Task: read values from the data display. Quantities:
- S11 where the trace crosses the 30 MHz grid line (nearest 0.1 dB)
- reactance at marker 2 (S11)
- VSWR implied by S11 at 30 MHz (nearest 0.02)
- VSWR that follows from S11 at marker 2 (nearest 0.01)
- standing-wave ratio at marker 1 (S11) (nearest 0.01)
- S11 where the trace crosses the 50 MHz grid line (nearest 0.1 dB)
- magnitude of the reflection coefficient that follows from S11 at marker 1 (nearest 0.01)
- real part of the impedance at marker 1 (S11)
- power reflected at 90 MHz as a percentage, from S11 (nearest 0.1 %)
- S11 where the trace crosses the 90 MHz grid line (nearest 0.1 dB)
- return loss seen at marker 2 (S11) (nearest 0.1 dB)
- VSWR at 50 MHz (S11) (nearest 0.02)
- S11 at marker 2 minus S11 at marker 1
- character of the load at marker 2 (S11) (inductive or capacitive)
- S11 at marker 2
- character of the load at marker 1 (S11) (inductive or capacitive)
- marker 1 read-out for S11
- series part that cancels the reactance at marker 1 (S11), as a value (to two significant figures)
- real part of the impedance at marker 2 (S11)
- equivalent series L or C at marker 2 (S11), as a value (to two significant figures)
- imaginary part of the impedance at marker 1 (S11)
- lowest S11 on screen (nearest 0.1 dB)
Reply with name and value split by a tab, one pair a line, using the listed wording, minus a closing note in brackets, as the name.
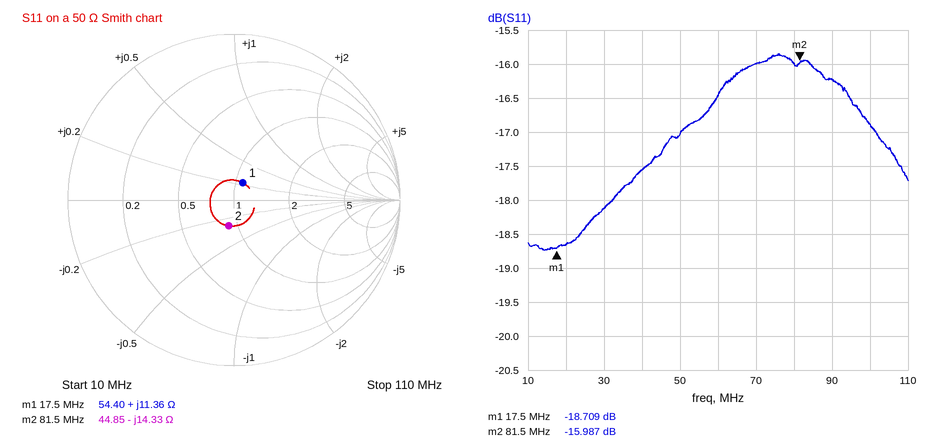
S11 where the trace crosses the 30 MHz grid line	-18.1 dB
reactance at marker 2	-14.33 Ω
VSWR implied by S11 at 30 MHz	1.28
VSWR that follows from S11 at marker 2	1.38
standing-wave ratio at marker 1 (S11)	1.26
S11 where the trace crosses the 50 MHz grid line	-17.0 dB
magnitude of the reflection coefficient that follows from S11 at marker 1	0.12
real part of the impedance at marker 1	54.40 Ω
power reflected at 90 MHz as a percentage, from S11	2.4 %
S11 where the trace crosses the 90 MHz grid line	-16.2 dB
return loss seen at marker 2 (S11)	16.0 dB
VSWR at 50 MHz (S11)	1.32
S11 at marker 2 minus S11 at marker 1	2.722 dB
character of the load at marker 2 (S11)	capacitive
S11 at marker 2	-15.987 dB
character of the load at marker 1 (S11)	inductive
marker 1 read-out for S11	-18.709 dB
series part that cancels the reactance at marker 1 (S11), as a value	800 pF
real part of the impedance at marker 2	44.85 Ω
equivalent series L or C at marker 2 (S11), as a value	140 pF
imaginary part of the impedance at marker 1	+11.36 Ω
lowest S11 on screen	-18.7 dB
